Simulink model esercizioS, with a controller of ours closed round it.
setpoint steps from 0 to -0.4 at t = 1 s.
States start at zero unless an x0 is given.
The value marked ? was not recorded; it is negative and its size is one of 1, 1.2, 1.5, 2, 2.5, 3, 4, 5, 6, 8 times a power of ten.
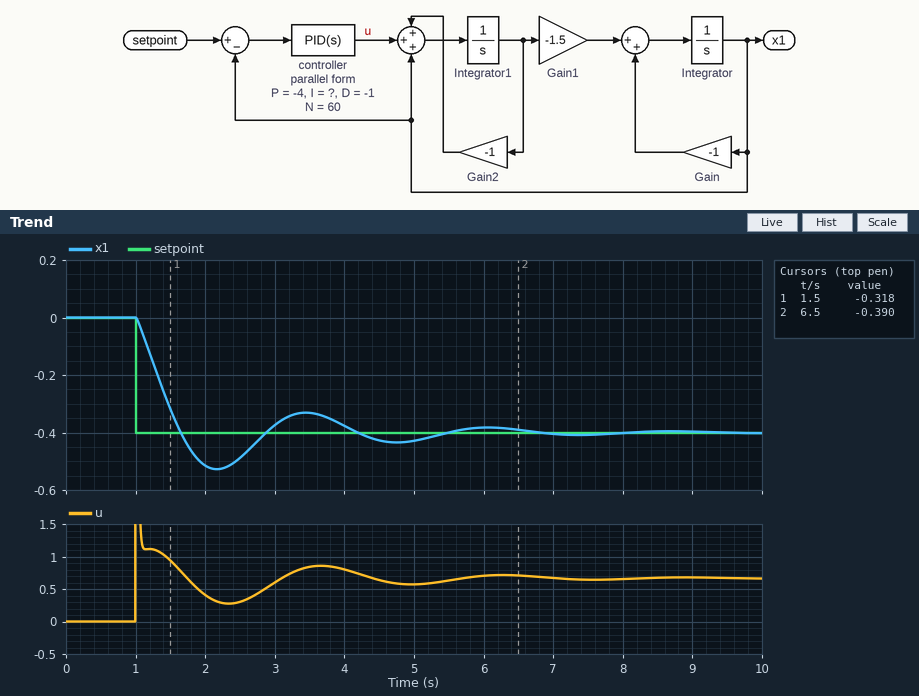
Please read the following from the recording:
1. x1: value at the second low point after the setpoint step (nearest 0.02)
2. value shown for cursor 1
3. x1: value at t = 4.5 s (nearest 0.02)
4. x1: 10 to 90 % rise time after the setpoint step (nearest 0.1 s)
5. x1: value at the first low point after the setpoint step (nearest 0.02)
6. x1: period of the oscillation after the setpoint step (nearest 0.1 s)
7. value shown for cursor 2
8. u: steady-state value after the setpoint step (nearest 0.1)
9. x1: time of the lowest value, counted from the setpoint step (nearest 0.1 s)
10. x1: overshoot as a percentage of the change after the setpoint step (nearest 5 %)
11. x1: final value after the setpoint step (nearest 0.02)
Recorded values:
-0.44
-0.318
-0.42
0.5 s
-0.52
2.6 s
-0.390
0.7
1.2 s
30 %
-0.40
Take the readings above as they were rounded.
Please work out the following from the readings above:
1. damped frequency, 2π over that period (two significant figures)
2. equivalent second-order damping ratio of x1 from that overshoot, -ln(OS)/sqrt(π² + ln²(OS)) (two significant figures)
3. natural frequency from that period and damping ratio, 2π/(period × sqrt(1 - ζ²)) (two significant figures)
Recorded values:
2.4 rad/s
0.36
2.6 rad/s
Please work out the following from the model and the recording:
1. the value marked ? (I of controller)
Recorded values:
-10
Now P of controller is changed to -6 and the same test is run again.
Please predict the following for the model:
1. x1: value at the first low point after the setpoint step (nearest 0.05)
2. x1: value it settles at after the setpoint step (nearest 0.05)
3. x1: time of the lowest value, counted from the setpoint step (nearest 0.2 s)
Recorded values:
-0.50
-0.40
1.0 s
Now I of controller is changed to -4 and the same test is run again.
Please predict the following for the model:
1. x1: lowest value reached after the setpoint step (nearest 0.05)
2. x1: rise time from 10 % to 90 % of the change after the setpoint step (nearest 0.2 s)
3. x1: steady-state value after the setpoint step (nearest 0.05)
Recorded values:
-0.40
0.6 s
-0.40
